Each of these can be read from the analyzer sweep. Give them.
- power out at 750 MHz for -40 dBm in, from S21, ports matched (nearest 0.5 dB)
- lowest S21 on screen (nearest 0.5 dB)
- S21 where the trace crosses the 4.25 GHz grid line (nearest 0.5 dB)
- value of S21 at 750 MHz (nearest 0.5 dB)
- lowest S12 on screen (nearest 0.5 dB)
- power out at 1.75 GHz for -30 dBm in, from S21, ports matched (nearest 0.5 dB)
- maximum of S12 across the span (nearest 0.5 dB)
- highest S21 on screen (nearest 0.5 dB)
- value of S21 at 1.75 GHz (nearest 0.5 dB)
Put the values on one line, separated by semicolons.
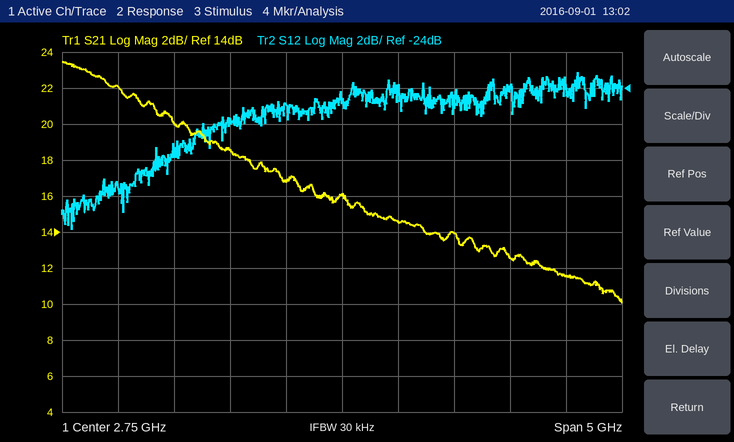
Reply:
-18.0 dBm; 10.0 dB; 12.5 dB; 22.0 dB; -32.0 dB; -11.5 dBm; -23.0 dB; 23.5 dB; 18.5 dB
